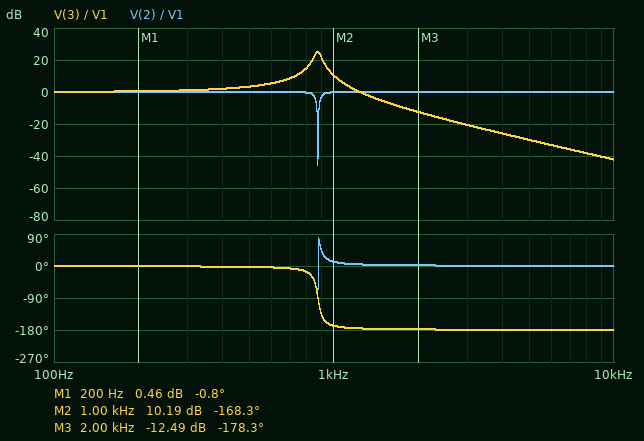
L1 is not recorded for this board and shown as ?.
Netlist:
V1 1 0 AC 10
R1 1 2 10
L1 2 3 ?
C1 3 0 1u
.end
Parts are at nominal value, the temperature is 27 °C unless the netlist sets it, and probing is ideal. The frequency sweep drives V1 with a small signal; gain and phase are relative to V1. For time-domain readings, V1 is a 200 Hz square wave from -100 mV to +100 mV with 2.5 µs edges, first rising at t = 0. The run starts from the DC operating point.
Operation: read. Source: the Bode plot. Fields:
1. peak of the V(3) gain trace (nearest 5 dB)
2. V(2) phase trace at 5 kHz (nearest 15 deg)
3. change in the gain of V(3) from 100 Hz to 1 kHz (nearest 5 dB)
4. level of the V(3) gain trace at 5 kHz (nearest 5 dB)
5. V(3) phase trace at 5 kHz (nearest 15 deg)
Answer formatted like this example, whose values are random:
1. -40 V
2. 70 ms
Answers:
1. 25 dB
2. 0 deg
3. 10 dB
4. -30 dB
5. -180 deg
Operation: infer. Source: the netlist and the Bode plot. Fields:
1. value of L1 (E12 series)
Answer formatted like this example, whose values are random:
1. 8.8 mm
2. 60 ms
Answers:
1. 33 mH
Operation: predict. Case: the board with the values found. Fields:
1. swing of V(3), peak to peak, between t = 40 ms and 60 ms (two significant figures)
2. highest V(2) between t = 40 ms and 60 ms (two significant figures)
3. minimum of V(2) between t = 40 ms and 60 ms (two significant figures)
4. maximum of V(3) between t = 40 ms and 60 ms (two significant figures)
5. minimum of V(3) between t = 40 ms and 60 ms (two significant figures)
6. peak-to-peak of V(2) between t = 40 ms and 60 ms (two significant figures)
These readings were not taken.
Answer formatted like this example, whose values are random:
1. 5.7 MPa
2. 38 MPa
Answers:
1. 460 mV
2. 110 mV
3. -110 mV
4. 230 mV
5. -230 mV
6. 210 mV
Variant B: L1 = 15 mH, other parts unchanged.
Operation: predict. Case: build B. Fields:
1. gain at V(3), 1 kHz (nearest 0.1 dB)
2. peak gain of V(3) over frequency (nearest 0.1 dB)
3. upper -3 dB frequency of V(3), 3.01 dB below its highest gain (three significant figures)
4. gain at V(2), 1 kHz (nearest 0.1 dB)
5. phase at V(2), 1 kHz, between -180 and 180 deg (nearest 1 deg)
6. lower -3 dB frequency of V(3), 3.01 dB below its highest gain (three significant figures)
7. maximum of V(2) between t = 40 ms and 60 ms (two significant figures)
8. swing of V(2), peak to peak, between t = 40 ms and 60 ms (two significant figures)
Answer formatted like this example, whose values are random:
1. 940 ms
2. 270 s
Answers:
1. 7.7 dB
2. 21.8 dB
3. 1.35 kHz
4. -0.1 dB
5. -9 deg
6. 1.24 kHz
7. 110 mV
8. 220 mV
